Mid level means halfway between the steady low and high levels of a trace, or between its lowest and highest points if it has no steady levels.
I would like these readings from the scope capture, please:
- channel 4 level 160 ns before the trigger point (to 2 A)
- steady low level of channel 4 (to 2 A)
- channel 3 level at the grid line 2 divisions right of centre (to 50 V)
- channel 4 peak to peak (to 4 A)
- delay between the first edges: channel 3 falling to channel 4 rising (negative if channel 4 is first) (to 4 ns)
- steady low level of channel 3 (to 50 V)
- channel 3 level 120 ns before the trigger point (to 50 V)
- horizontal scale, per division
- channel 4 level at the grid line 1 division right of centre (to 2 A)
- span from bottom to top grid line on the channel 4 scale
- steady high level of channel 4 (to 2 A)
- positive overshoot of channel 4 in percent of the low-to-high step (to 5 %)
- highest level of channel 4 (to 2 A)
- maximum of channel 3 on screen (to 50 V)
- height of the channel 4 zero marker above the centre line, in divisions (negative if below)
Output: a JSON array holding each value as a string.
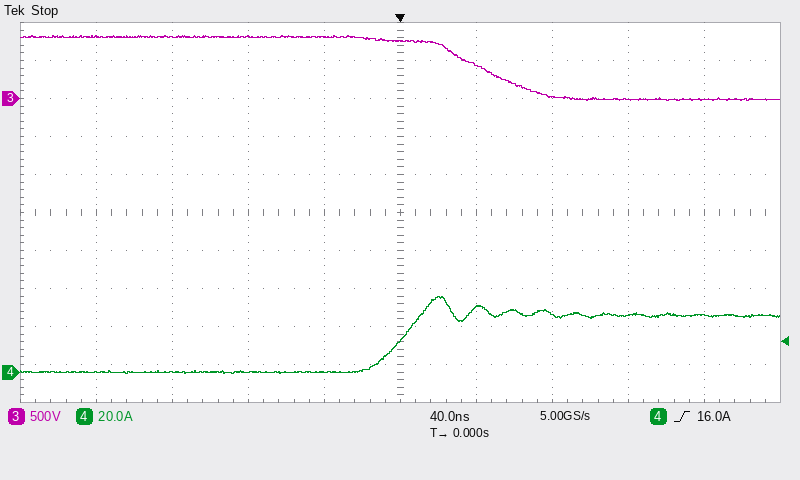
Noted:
["0 A", "0 A", "0 V", "40 A", "-44 ns", "0 V", "800 V", "40 ns", "34 A", "200 A", "30 A", "35 %", "40 A", "850 V", "-4.2 div"]
